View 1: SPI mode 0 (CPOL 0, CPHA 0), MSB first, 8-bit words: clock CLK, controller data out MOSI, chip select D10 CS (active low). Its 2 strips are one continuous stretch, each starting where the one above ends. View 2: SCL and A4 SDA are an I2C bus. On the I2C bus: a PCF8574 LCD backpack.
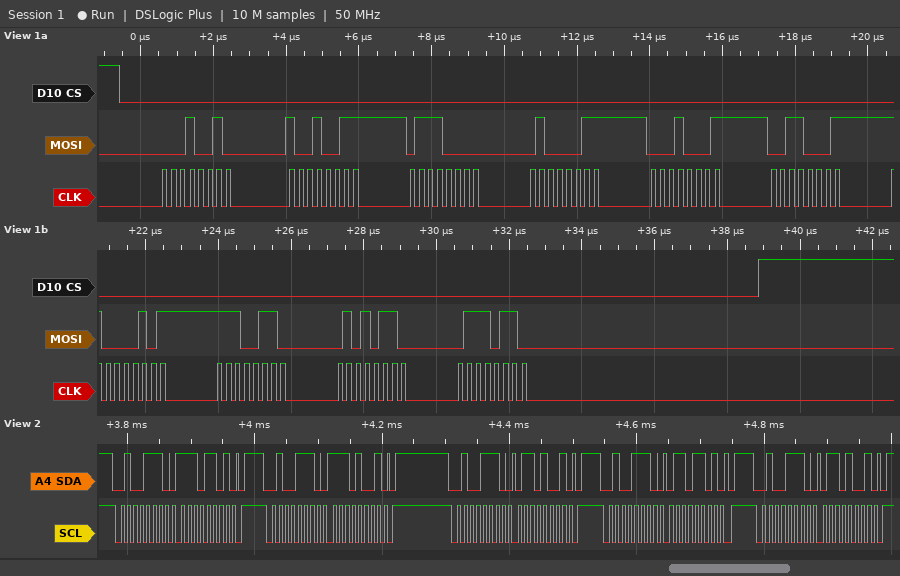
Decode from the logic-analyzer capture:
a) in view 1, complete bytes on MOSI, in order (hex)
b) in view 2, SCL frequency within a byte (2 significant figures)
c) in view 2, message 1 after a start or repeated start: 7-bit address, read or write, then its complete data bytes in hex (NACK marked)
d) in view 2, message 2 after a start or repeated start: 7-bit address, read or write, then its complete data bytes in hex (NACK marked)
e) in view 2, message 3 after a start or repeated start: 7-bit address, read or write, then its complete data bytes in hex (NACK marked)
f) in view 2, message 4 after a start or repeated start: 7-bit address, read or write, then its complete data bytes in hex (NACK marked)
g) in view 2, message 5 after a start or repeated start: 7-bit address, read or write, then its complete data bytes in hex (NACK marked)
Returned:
0x12 0x93 0x70 0x43 0x11 0x31 0x85 0xE6 0x56 0x76
100 kHz
0x27 write: ED
0x27 write: E9
0x27 write: 69
0x27 write: 6D
0x27 write: 69
